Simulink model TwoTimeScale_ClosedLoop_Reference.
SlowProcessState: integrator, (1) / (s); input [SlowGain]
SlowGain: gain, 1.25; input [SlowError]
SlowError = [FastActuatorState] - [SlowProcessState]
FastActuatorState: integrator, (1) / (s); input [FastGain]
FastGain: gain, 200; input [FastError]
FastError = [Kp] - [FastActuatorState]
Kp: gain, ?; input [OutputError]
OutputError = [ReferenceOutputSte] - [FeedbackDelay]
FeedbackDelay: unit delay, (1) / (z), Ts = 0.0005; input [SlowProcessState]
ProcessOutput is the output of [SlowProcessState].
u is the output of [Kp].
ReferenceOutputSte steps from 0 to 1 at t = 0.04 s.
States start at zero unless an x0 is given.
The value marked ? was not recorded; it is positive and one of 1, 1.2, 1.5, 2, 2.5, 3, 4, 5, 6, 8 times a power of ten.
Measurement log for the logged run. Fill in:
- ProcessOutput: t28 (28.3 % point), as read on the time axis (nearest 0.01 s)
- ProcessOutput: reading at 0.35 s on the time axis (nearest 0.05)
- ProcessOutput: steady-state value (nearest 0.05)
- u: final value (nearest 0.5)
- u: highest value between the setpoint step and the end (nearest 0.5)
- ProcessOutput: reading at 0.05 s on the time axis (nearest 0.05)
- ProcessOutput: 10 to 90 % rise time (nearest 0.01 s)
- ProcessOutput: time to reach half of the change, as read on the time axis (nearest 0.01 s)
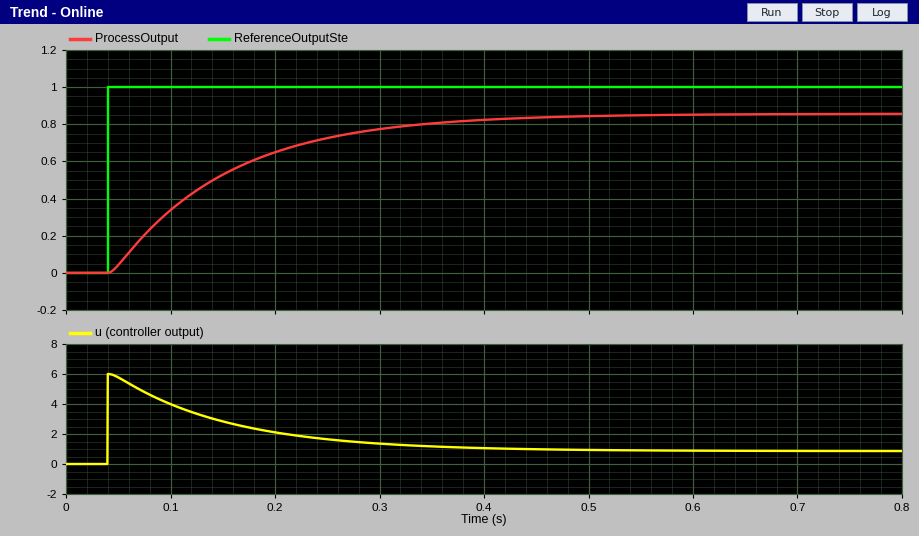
0.08 s
0.80
0.85
1.0
6.0
0.05
0.24 s
0.12 s
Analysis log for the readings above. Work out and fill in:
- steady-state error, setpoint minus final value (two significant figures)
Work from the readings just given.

0.15
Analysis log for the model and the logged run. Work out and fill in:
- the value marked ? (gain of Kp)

6
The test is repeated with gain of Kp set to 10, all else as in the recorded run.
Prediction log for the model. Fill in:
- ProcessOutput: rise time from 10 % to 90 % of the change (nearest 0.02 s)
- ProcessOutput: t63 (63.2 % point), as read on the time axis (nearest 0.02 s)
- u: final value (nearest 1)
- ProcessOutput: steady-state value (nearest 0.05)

0.14 s
0.12 s
1
0.90
